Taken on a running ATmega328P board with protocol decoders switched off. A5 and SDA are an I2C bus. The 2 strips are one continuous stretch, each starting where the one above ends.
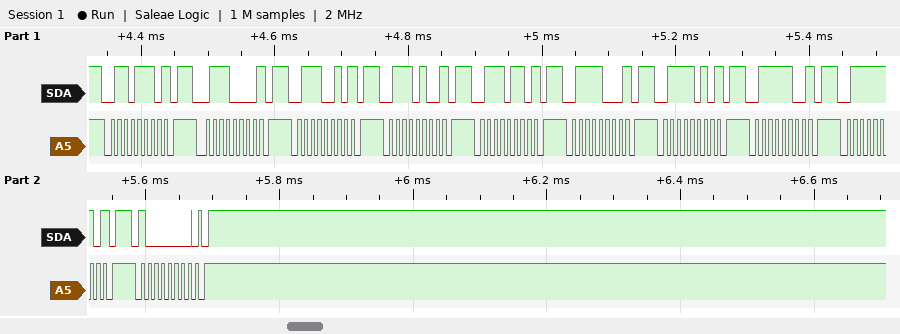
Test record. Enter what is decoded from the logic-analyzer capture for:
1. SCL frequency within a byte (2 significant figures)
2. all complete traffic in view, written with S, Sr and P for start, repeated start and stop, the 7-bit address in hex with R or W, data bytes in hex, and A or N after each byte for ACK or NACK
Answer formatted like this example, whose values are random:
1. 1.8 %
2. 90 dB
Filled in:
1. 100 kHz
2. S 37W N P S 38W N P S 39W N P S 3AW N P S 3BW N P S 3CW N P S 3DW N P S 3EW N P S 3FW N P S 40W A P
